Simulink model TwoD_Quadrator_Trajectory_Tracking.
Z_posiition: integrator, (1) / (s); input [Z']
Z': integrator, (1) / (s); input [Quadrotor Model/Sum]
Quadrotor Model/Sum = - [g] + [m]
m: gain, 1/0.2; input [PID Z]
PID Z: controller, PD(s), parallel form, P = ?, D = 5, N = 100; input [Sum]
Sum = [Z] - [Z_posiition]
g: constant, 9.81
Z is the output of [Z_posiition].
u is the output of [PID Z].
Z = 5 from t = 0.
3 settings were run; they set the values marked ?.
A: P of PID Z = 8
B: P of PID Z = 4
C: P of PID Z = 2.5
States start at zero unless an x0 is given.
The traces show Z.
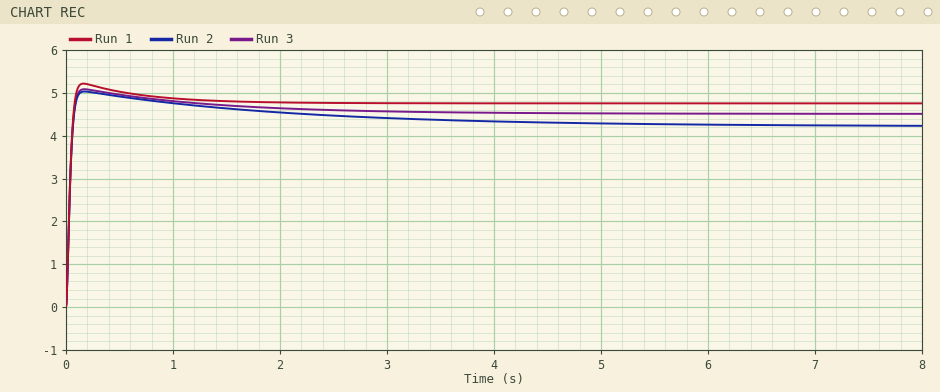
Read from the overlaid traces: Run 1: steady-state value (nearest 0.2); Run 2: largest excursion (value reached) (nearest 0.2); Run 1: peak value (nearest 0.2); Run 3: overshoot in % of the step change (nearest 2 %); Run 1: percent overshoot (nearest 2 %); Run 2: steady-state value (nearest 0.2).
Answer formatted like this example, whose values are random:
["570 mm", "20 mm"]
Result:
["4.8", "5.0", "5.2", "12 %", "10 %", "4.2"]
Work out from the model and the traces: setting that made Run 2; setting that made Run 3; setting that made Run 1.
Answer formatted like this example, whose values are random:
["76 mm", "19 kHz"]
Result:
["C", "B", "A"]
